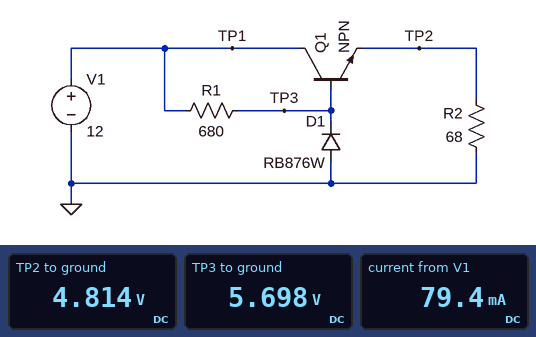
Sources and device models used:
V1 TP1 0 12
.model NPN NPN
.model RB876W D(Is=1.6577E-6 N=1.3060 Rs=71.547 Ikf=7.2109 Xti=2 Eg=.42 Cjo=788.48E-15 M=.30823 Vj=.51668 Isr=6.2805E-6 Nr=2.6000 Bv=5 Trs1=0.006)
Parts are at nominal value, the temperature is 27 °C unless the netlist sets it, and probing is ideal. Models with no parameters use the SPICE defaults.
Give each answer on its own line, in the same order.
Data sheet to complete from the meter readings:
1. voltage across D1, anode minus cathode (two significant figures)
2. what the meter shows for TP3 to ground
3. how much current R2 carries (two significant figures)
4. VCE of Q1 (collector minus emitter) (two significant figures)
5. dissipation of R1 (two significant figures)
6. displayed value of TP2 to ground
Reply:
-5.7 V
5.698 V
71 mA
7.2 V
58 mW
4.814 V
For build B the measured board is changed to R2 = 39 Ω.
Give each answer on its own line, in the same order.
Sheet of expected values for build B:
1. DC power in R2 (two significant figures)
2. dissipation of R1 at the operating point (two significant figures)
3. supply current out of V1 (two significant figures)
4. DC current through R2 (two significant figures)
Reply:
580 mW
59 mW
130 mA
120 mA
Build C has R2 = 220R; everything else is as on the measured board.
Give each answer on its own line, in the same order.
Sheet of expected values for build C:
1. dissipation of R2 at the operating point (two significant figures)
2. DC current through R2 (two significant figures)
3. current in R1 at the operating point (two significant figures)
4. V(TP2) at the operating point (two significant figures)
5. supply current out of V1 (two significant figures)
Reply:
110 mW
22 mA
9.2 mA
4.9 V
31 mA
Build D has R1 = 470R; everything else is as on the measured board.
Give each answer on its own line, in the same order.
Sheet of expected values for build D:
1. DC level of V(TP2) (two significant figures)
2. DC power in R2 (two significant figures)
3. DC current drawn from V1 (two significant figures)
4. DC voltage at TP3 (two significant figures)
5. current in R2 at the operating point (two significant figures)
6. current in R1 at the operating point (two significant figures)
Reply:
5.1 V
380 mW
87 mA
6.0 V
75 mA
13 mA
